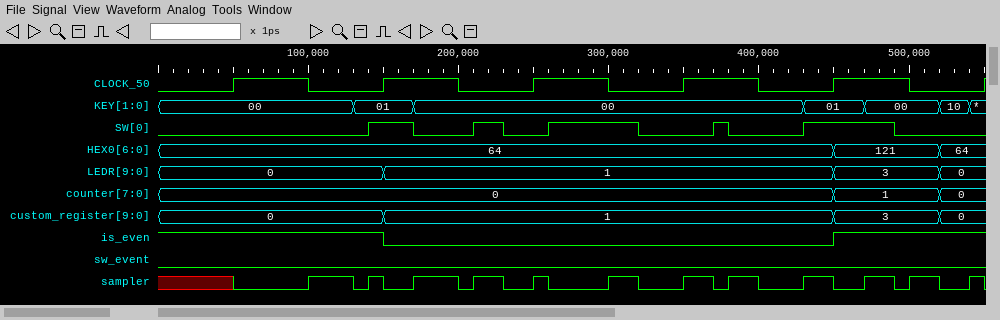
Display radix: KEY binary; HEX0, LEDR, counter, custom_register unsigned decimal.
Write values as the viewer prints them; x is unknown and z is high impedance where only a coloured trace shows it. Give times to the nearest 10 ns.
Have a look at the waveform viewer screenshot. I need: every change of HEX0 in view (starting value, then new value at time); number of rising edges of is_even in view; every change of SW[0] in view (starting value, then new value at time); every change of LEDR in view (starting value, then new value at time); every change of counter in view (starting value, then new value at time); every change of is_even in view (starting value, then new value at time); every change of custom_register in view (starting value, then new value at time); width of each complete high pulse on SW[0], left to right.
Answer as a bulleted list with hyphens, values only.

- 64, 121 at 450 ns, 64 at 520 ns
- 1
- 0, 1 at 140 ns, 0 at 170 ns, 1 at 210 ns, 0 at 230 ns, 1 at 260 ns, 0 at 320 ns, 1 at 370 ns, 0 at 380 ns, 1 at 430 ns, 0 at 490 ns
- 0, 1 at 150 ns, 3 at 450 ns, 0 at 520 ns
- 0, 1 at 450 ns, 0 at 520 ns
- 1, 0 at 150 ns, 1 at 450 ns
- 0, 1 at 150 ns, 3 at 450 ns, 0 at 520 ns
- 30 ns, 20 ns, 60 ns, 10 ns, 60 ns
